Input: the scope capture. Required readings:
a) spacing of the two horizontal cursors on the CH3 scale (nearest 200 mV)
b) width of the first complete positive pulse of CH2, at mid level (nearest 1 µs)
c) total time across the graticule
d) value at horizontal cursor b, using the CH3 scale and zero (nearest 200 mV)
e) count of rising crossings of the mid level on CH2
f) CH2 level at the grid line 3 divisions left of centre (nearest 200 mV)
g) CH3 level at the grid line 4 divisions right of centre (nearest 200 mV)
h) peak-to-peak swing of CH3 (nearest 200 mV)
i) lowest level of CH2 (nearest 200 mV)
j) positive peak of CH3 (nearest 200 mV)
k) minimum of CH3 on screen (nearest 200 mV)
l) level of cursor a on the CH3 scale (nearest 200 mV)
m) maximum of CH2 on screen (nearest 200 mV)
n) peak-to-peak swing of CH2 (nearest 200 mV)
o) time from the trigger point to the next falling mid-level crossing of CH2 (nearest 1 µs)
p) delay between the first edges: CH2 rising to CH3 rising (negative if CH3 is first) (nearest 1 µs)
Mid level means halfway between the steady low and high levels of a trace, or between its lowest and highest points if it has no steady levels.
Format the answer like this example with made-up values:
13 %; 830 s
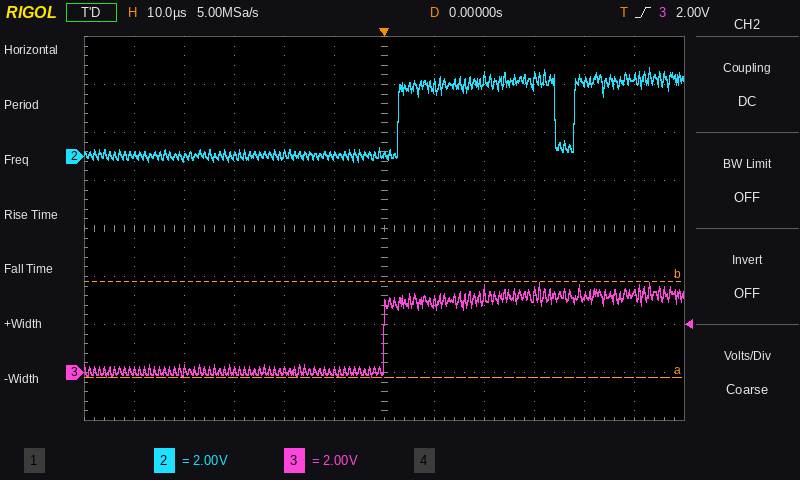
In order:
4.0 V; 31 µs; 120 µs; 3.8 V; 2; 0.0 V; 3.2 V; 4.0 V; -200 mV; 3.8 V; -200 mV; -200 mV; 3.8 V; 4.0 V; 34 µs; -3 µs
